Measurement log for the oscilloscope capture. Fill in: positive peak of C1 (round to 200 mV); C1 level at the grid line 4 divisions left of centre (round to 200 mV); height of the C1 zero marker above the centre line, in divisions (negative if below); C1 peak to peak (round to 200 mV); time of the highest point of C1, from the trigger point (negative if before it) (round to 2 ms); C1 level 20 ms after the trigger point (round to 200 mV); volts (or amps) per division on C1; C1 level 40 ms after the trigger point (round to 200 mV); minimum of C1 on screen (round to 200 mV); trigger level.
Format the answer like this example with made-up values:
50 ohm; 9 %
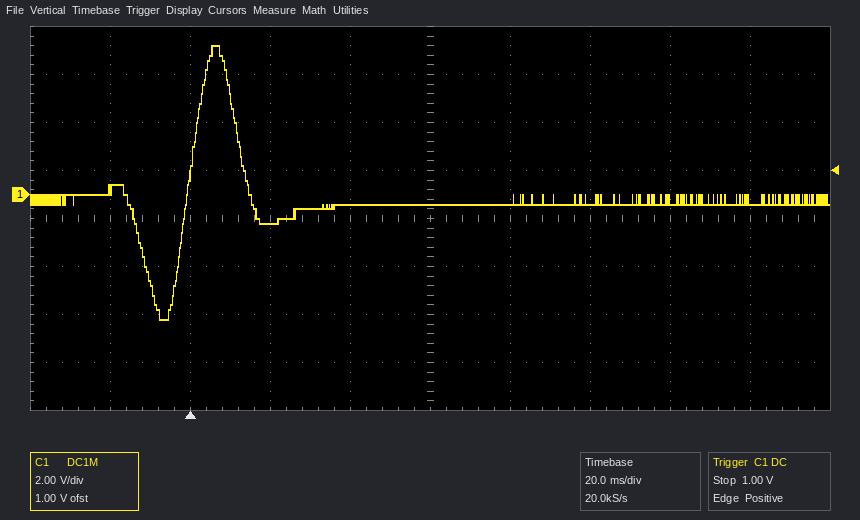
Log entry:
6.2 V; 200 mV; +0.5 div; 11.4 V; +6 ms; -1.2 V; 2 V; -400 mV; -5.2 V; 1.00 V
